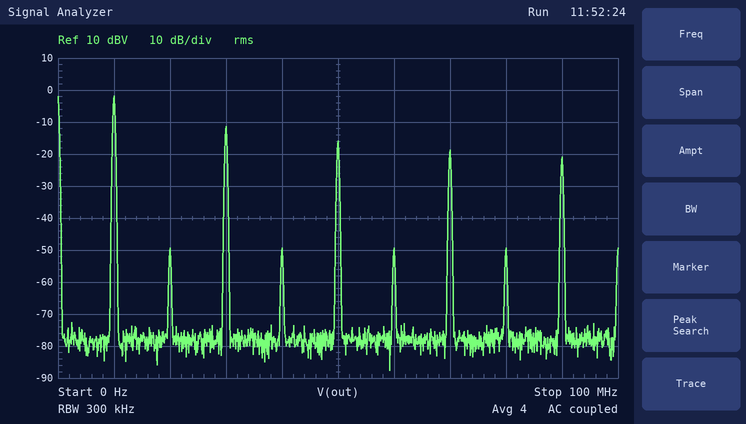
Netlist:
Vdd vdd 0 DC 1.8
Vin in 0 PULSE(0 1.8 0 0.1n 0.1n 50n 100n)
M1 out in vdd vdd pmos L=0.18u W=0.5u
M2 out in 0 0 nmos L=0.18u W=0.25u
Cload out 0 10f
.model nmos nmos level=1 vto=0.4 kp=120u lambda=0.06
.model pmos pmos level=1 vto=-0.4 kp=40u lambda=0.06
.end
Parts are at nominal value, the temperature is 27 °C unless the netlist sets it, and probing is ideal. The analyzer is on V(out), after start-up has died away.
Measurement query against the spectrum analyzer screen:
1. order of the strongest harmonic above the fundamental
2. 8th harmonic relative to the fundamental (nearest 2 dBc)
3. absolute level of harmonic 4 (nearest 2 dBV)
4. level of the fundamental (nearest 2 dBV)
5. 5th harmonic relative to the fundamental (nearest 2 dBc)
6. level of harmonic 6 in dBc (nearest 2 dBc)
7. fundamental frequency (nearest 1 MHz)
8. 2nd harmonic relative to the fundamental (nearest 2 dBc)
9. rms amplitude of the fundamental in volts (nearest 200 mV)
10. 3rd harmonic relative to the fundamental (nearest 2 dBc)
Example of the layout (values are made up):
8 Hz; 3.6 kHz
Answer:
3; -48 dBc; -50 dBV; -2 dBV; -14 dBc; -48 dBc; 10 MHz; -48 dBc; 800 mV; -10 dBc
